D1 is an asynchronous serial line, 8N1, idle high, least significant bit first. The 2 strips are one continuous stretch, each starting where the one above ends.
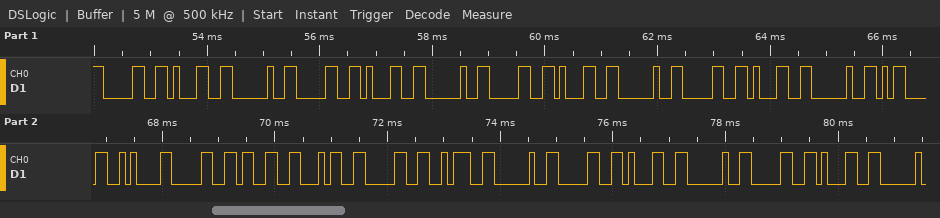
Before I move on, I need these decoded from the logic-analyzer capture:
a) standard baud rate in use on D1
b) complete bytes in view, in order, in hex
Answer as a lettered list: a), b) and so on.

a) 9600 baud
b) 30 31 20 30 31 20 30 31 20 30 31 20 0D 0A 30 33 34 30 3A 20 30 31 20 30 31
